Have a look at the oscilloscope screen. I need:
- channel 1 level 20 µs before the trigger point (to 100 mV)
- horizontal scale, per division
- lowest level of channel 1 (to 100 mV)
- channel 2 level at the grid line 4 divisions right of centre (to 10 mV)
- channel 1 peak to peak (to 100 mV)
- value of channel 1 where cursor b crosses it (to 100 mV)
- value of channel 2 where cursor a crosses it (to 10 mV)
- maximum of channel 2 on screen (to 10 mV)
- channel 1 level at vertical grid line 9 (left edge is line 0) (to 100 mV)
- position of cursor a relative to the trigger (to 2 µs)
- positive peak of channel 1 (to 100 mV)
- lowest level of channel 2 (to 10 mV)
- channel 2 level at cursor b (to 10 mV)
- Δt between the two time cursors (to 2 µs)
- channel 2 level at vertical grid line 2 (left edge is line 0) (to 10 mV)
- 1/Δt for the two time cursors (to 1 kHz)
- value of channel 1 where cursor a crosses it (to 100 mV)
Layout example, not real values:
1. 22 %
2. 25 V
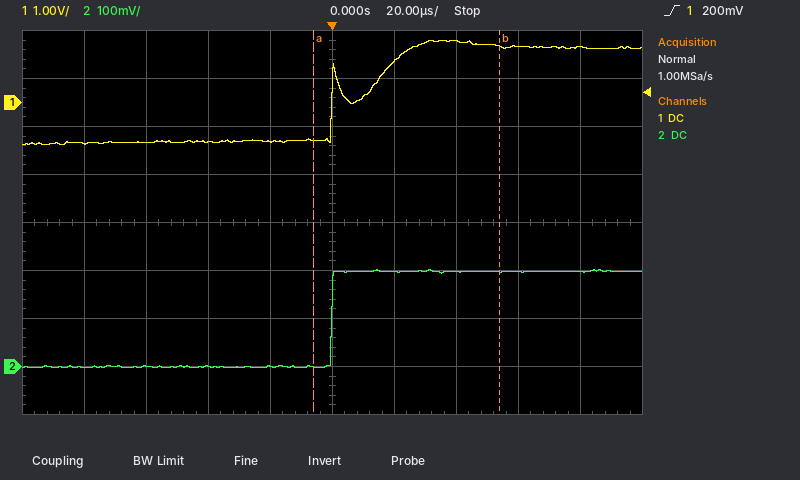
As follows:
1. -800 mV
2. 20 µs
3. -900 mV
4. 200 mV
5. 2.2 V
6. 1.2 V
7. 0 mV
8. 200 mV
9. 1.2 V
10. -6 µs
11. 1.3 V
12. 0 mV
13. 200 mV
14. 60 µs
15. 0 mV
16. 17 kHz
17. -800 mV
